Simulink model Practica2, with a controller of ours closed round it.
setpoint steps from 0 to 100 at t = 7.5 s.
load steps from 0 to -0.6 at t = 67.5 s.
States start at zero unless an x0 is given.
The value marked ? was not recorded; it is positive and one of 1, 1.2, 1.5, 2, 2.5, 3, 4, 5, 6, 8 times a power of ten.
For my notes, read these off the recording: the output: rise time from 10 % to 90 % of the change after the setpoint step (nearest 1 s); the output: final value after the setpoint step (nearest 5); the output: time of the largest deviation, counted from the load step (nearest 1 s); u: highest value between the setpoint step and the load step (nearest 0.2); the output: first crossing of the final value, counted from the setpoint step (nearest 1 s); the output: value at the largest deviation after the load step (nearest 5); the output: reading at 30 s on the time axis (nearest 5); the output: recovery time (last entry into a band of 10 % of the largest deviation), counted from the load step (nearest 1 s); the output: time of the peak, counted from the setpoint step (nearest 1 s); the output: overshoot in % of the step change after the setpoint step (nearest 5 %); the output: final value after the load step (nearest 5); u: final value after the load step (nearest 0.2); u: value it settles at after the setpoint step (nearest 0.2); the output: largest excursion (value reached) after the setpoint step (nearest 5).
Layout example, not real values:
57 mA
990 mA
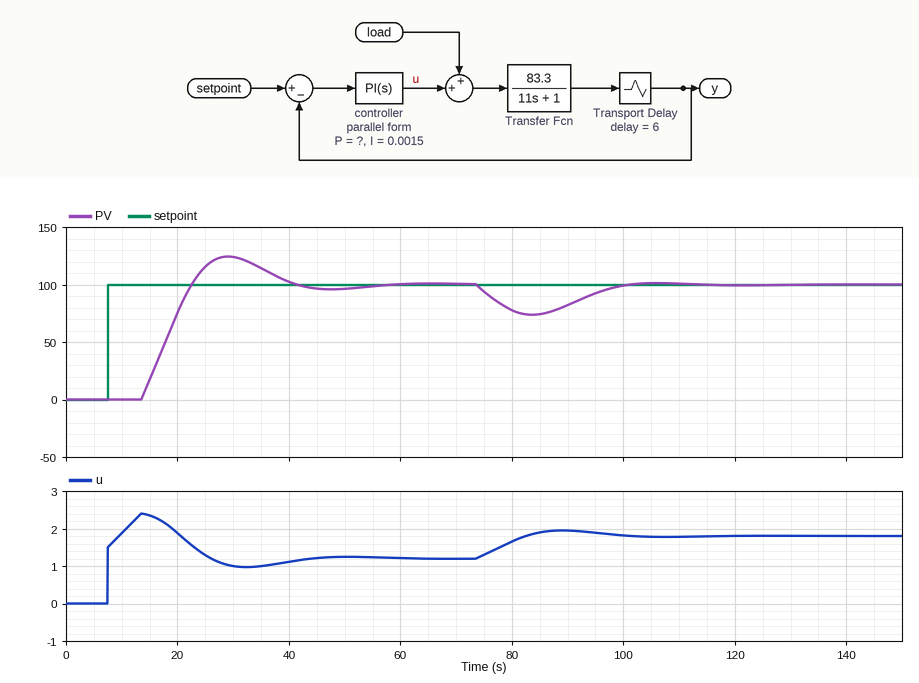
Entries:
7 s
100
16 s
2.4
15 s
75
125
31 s
22 s
25 %
100
1.8
1.2
125
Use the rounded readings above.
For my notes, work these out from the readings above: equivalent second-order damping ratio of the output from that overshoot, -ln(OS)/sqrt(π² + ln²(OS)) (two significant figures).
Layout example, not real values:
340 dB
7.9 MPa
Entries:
0.40
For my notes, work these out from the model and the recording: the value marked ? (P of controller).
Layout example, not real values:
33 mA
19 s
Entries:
0.015
